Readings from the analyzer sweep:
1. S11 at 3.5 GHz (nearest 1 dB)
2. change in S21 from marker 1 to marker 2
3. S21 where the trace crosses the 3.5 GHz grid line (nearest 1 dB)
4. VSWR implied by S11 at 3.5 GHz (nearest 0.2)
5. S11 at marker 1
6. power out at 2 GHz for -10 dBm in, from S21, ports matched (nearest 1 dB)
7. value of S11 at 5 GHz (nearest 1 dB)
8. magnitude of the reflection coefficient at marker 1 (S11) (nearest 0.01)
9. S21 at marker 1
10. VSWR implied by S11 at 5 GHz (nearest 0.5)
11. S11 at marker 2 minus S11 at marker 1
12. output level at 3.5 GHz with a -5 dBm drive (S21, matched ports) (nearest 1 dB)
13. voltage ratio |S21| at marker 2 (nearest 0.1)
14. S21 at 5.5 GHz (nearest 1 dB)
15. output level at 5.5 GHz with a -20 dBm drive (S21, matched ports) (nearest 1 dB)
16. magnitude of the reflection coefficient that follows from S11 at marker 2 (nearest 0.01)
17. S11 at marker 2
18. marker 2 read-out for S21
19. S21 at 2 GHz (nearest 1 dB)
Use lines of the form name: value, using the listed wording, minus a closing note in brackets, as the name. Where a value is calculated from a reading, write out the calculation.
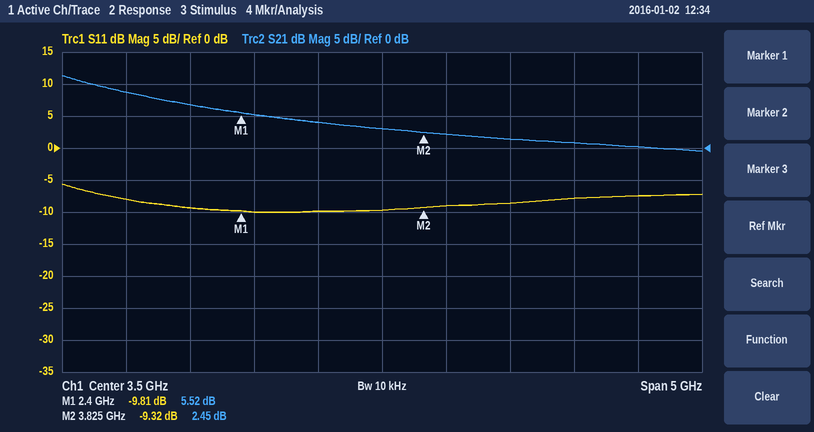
S11 at 3.5 GHz: -10 dB
change in S21 from marker 1 to marker 2: 2.45 − (5.52) = -3.07 dB
S21 where the trace crosses the 3.5 GHz grid line: 3 dB
VSWR implied by S11 at 3.5 GHz: |Γ| = 10^(-10/20) = 0.3162; VSWR = (1 + 0.3162)/(1 − 0.3162) ≈ 1.92, so 2.0 to the nearest 0.2
S11 at marker 1: -9.81 dB
power out at 2 GHz for -10 dBm in, from S21, ports matched: -10 dBm + (7 dB) = -3 dBm
value of S11 at 5 GHz: -8 dB
magnitude of the reflection coefficient at marker 1 (S11): 10^(-9.81/20) ≈ 0.32
S21 at marker 1: 5.52 dB
VSWR implied by S11 at 5 GHz: |Γ| = 10^(-8/20) = 0.3981; VSWR = (1 + 0.3981)/(1 − 0.3981) ≈ 2.32, so 2.5 to the nearest 0.5
S11 at marker 2 minus S11 at marker 1: -9.32 − (-9.81) = 0.49 dB
output level at 3.5 GHz with a -5 dBm drive (S21, matched ports): -5 dBm + (3 dB) = -2 dBm
voltage ratio |S21| at marker 2: 10^(2.45/20) ≈ 1.3
S21 at 5.5 GHz: 0 dB
output level at 5.5 GHz with a -20 dBm drive (S21, matched ports): -20 dBm + (0 dB) = -20 dBm
magnitude of the reflection coefficient that follows from S11 at marker 2: 10^(-9.32/20) ≈ 0.34
S11 at marker 2: -9.32 dB
marker 2 read-out for S21: 2.45 dB
S21 at 2 GHz: 7 dB
